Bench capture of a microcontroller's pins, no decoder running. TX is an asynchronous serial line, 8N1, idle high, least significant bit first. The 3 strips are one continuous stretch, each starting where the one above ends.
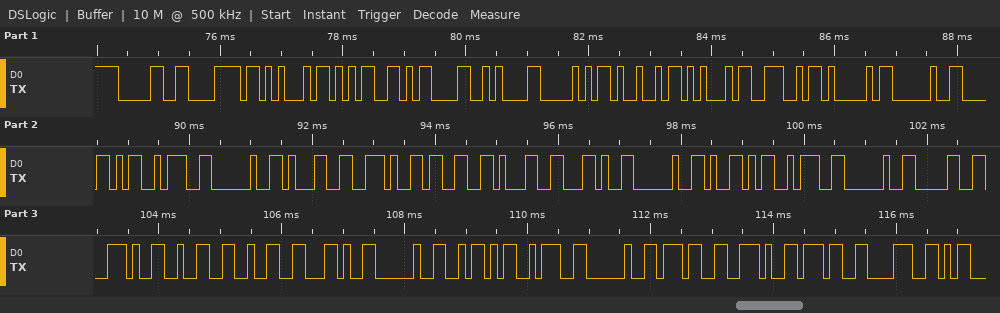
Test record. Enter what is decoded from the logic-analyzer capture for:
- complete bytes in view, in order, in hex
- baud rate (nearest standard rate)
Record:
0x30 0x78 0x45 0x35 0x0D 0x0A 0x50 0x49 0x45 0x4E 0x41 0x20 0x58 0x3A 0x20 0x31 0x2E 0x33 0x31 0x2C 0x20 0x59 0x3A 0x20 0x30 0x2E 0x32 0x32 0x2C 0x20 0x5A 0x3A 0x20 0x37 0x2E 0x37 0x38
9600 baud
